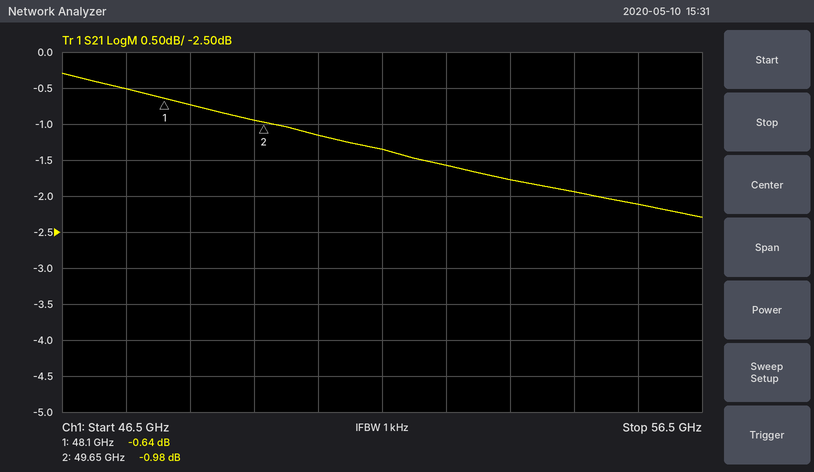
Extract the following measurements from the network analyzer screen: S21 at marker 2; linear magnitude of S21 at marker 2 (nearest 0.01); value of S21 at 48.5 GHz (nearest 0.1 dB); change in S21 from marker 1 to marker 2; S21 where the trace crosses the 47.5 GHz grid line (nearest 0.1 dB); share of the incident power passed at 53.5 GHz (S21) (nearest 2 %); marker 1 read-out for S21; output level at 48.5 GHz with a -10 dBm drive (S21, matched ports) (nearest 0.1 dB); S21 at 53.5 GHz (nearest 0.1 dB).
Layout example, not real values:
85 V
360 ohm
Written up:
-0.98 dB
0.89
-0.7 dB
-0.34 dB
-0.5 dB
66 %
-0.64 dB
-10.7 dBm
-1.8 dB
